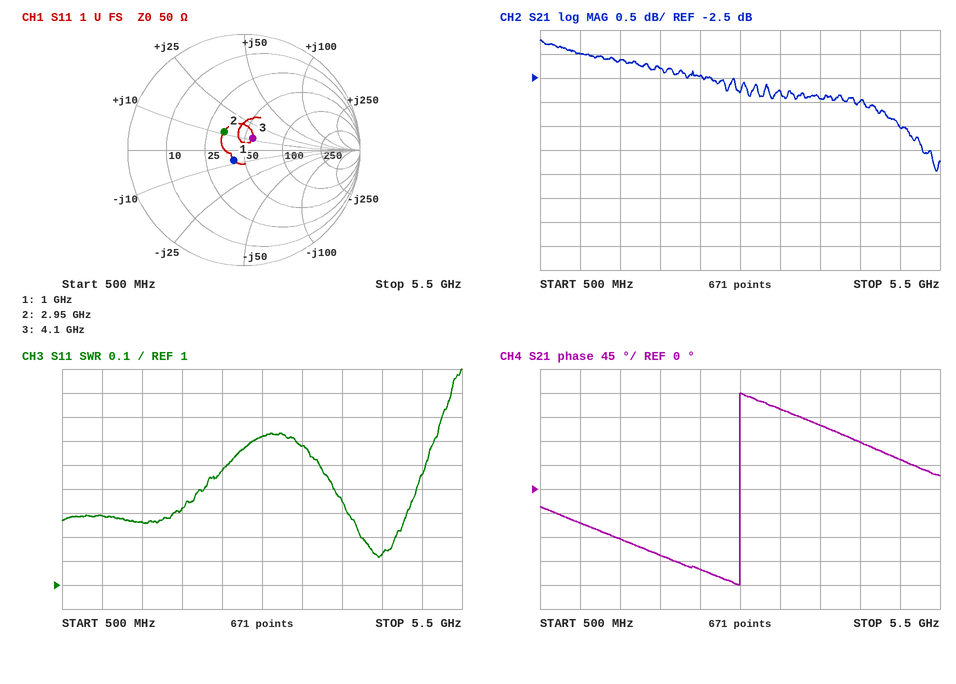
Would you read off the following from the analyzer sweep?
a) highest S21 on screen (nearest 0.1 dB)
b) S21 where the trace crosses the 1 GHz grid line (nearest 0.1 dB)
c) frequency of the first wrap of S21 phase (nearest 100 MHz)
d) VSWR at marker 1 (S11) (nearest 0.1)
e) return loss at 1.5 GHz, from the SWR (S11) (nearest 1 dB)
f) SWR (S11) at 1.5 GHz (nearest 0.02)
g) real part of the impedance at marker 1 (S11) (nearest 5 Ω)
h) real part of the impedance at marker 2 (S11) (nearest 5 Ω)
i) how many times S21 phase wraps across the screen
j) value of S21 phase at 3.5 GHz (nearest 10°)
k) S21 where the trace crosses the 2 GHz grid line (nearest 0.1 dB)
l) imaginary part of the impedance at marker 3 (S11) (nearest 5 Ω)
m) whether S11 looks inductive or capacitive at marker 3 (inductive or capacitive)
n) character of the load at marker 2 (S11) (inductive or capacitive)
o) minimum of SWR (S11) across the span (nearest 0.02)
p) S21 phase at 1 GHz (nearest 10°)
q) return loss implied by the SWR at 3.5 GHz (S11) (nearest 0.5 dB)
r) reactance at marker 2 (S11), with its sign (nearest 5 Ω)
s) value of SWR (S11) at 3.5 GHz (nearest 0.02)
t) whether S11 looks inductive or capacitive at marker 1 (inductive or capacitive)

-1.7 dB
-2.0 dB
3.0 GHz
1.3
19 dB
1.26
40 Ω
35 Ω
1
150°
-2.3 dB
+10 Ω
inductive
inductive
1.12
-60°
13.0 dB
+10 Ω
1.58
capacitive
